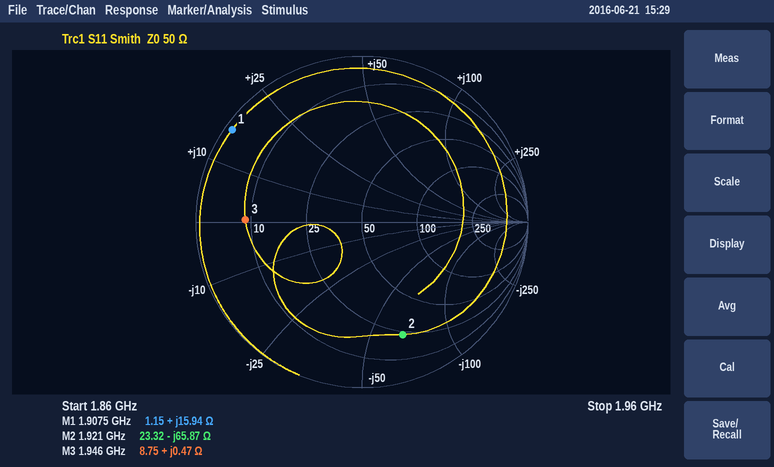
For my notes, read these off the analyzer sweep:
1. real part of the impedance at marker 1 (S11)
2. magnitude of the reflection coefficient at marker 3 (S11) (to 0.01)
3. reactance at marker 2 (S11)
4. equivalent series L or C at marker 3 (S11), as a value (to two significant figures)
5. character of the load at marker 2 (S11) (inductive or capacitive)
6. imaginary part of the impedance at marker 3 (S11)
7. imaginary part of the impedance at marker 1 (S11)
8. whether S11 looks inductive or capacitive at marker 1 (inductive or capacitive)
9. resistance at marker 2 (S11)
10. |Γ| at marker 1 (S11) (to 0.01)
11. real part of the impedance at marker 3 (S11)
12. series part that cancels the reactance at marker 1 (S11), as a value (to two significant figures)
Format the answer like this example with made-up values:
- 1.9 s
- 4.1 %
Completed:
- 1.15 Ω
- 0.70
- -65.87 Ω
- 38 pH
- capacitive
- +0.47 Ω
- +15.94 Ω
- inductive
- 23.32 Ω
- 0.96
- 8.75 Ω
- 5.2 pF
